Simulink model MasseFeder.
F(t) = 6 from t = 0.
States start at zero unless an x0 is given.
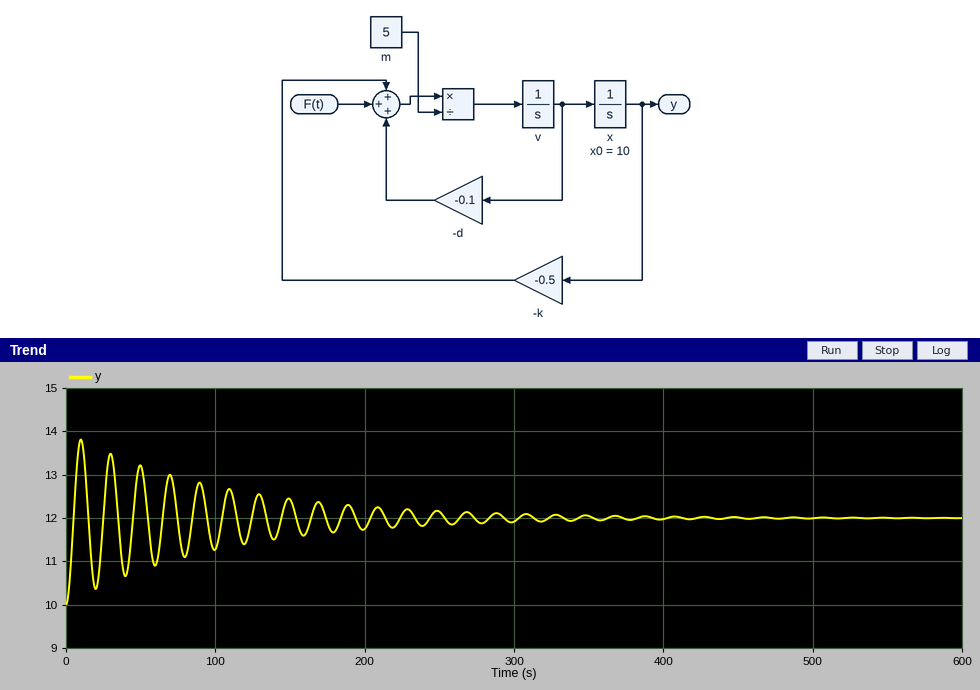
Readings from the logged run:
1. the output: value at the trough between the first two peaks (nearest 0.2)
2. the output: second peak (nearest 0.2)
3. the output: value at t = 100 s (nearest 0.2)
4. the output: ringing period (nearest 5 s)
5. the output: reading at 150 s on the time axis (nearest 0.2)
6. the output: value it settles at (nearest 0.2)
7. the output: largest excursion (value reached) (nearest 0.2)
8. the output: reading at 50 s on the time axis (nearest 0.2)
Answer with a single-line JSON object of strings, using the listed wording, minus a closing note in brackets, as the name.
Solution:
{"the output: value at the trough between the first two peaks": "10.4", "the output: second peak": "13.4", "the output: value at t = 100 s": "11.2", "the output: ringing period": "20 s", "the output: reading at 150 s on the time axis": "12.4", "the output: value it settles at": "12.0", "the output: largest excursion (value reached)": "13.8", "the output: reading at 50 s on the time axis": "13.2"}
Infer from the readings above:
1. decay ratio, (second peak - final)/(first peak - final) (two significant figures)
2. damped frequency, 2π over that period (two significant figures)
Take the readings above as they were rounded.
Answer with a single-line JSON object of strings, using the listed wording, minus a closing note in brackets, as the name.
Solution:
{"decay ratio, (second peak - final)/(first peak - final)": "0.78", "damped frequency, 2π over that period": "0.31 rad/s"}
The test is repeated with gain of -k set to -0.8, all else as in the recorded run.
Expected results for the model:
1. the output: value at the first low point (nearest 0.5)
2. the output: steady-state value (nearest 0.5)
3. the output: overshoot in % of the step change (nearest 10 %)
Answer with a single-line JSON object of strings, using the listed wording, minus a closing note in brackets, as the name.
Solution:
{"the output: value at the first low point": "5.0", "the output: steady-state value": "7.5", "the output: overshoot in % of the step change": "90 %"}
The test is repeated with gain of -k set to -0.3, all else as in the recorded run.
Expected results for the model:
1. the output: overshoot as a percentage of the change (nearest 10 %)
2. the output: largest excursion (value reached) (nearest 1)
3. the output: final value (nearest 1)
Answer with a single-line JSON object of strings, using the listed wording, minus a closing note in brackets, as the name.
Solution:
{"the output: overshoot as a percentage of the change": "90 %", "the output: largest excursion (value reached)": "29", "the output: final value": "20"}
